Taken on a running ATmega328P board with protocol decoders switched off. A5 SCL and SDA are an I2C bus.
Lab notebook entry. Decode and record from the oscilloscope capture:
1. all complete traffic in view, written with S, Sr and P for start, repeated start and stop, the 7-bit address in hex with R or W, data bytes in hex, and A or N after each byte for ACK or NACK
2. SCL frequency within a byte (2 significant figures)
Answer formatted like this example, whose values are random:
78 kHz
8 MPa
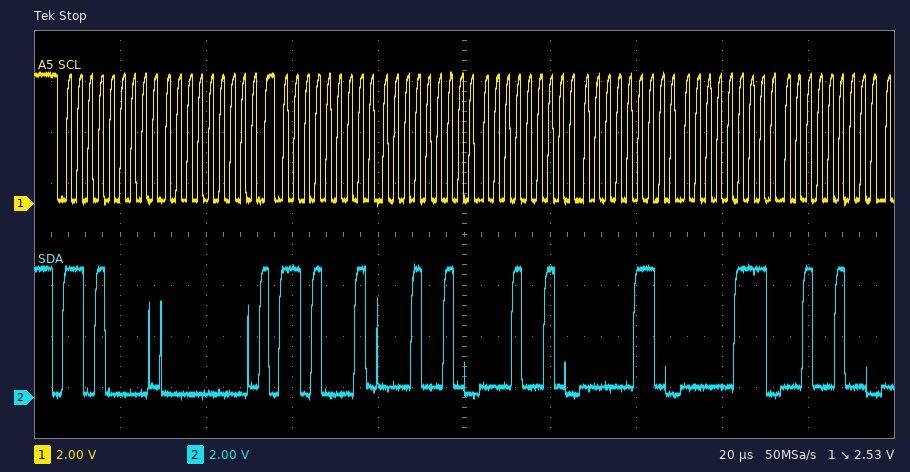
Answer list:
S 68W A 00 A Sr 68R A 12 A 12 A 06 A 07 A 24 A
400 kHz
